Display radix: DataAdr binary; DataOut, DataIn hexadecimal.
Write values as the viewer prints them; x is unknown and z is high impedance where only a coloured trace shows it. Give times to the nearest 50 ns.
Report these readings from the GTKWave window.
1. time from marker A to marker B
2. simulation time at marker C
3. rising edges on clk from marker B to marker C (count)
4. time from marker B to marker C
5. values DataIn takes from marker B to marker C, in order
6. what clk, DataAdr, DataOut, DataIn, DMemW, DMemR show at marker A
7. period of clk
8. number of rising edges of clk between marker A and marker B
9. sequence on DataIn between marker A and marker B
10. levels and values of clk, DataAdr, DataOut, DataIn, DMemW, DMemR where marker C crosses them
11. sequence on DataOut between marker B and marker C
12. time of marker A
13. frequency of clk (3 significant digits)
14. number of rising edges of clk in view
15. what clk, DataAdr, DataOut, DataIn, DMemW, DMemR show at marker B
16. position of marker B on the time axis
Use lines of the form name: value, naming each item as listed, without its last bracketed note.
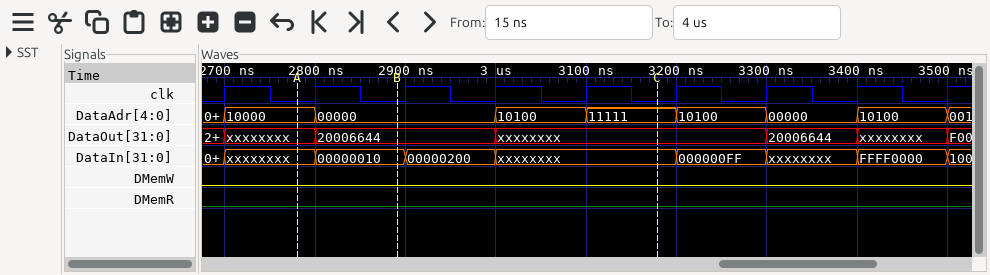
time from marker A to marker B: 100 ns
simulation time at marker C: 3200 ns
rising edges on clk from marker B to marker C: 3
time from marker B to marker C: 300 ns
values DataIn takes from marker B to marker C, in order: 00000010, 00000200, xxxxxxxx
what clk, DataAdr, DataOut, DataIn, DMemW, DMemR show at marker A: clk=0, DataAdr=10000, DataOut=xxxxxxxx, DataIn=xxxxxxxx, DMemW=0, DMemR=0
period of clk: 100 ns
number of rising edges of clk between marker A and marker B: 1
sequence on DataIn between marker A and marker B: xxxxxxxx, 00000010
levels and values of clk, DataAdr, DataOut, DataIn, DMemW, DMemR where marker C crosses them: clk=0, DataAdr=11111, DataOut=xxxxxxxx, DataIn=xxxxxxxx, DMemW=0, DMemR=0
sequence on DataOut between marker B and marker C: 20006644, xxxxxxxx
time of marker A: 2800 ns
frequency of clk: 10.0 MHz
number of rising edges of clk in view: 9
what clk, DataAdr, DataOut, DataIn, DMemW, DMemR show at marker B: clk=0, DataAdr=00000, DataOut=20006644, DataIn=00000010, DMemW=0, DMemR=0
position of marker B on the time axis: 2900 ns
